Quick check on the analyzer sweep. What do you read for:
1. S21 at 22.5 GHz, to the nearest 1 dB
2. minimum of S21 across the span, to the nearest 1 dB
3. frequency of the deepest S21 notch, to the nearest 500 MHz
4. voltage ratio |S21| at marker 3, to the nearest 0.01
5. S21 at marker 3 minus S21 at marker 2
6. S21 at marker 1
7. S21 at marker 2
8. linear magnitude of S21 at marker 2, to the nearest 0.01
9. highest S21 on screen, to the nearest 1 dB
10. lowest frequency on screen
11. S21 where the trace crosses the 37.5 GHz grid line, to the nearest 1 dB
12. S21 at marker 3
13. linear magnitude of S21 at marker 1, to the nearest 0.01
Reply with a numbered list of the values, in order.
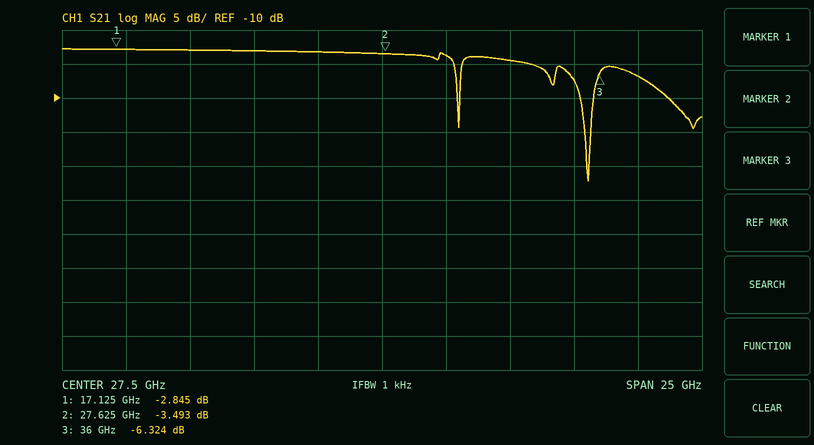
1. -3 dB
2. -22 dB
3. 35.5 GHz
4. 0.48
5. -2.831 dB
6. -2.845 dB
7. -3.493 dB
8. 0.67
9. -3 dB
10. 15 GHz
11. -7 dB
12. -6.324 dB
13. 0.72
